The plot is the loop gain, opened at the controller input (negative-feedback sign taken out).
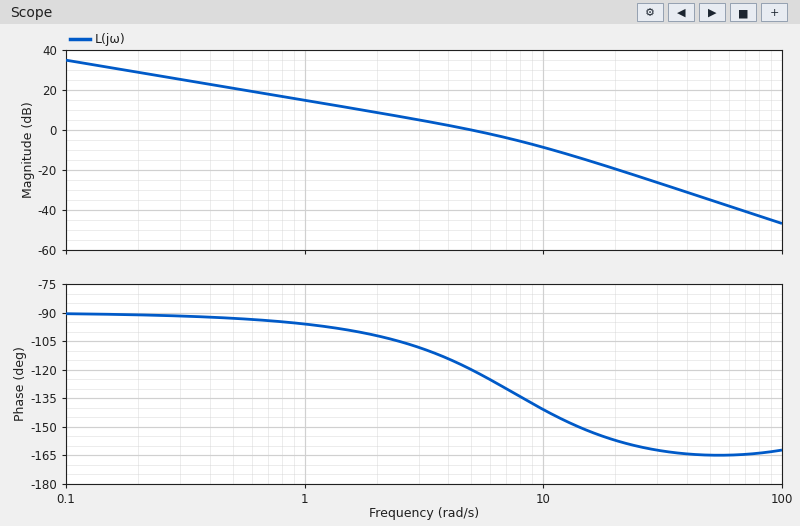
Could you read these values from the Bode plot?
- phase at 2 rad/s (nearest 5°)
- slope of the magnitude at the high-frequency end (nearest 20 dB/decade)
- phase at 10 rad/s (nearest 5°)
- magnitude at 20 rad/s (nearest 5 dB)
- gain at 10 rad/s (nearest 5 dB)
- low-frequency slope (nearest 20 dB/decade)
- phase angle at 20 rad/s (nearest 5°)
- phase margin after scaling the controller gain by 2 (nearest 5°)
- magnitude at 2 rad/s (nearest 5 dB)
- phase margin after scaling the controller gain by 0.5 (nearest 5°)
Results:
-100°
-40 dB/decade
-140°
-20 dB
-10 dB
-20 dB/decade
-155°
45°
10 dB
75°
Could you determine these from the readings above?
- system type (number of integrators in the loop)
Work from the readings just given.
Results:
1
